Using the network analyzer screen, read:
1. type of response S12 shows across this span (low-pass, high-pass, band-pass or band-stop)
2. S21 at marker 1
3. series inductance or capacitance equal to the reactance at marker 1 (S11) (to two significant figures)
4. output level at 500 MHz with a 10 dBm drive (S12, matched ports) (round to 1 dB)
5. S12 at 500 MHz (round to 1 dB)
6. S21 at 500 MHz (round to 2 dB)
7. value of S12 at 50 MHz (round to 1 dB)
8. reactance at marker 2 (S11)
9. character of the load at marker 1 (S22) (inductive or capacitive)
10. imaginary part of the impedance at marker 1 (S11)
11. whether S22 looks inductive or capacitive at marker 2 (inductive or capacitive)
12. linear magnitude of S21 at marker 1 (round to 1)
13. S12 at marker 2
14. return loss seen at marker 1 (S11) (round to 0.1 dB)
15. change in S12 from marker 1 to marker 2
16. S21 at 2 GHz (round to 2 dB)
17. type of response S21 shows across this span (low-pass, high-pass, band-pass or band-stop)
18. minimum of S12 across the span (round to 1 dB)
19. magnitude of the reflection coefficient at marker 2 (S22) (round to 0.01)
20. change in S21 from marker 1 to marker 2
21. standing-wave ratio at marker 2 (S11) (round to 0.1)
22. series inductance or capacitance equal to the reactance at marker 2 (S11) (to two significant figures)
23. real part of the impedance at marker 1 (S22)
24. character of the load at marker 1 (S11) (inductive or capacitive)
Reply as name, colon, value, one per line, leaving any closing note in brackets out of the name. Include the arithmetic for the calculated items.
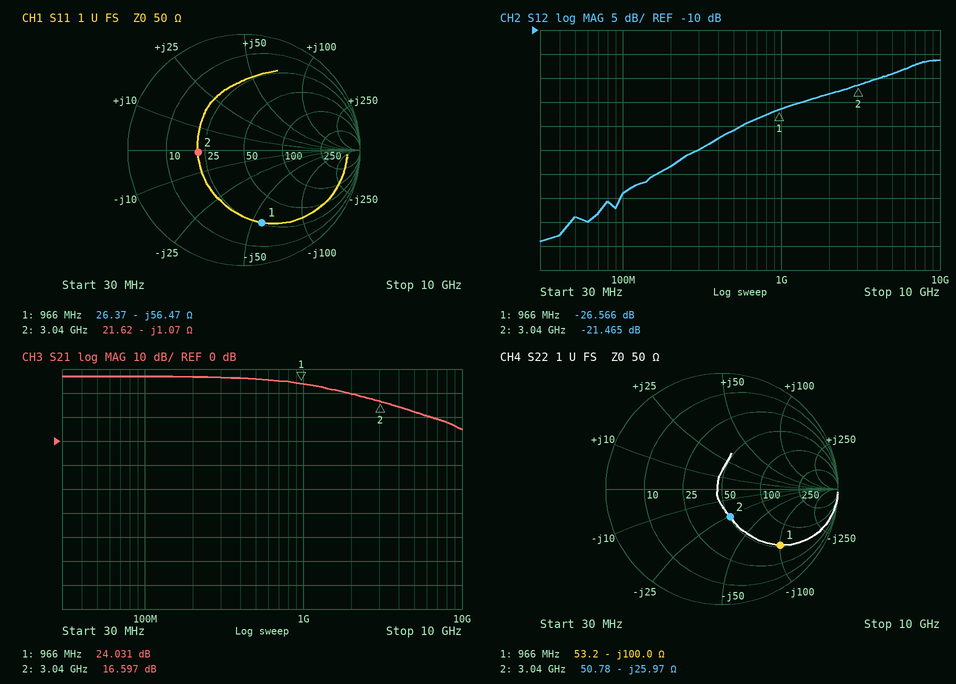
type of response S12 shows across this span: high-pass
S21 at marker 1: 24.031 dB
series inductance or capacitance equal to the reactance at marker 1 (S11): C = 1/(2π × 966 MHz × 56.47 Ω) ≈ 2.9 pF
output level at 500 MHz with a 10 dBm drive (S12, matched ports): 10 dBm + (-31 dB) = -21 dBm
S12 at 500 MHz: -31 dB
S21 at 500 MHz: 26 dB
value of S12 at 50 MHz: -49 dB
reactance at marker 2: -1.07 Ω
character of the load at marker 1 (S22): capacitive
imaginary part of the impedance at marker 1: -56.47 Ω
whether S22 looks inductive or capacitive at marker 2: capacitive
linear magnitude of S21 at marker 1: 10^(24.031/20) ≈ 16
S12 at marker 2: -21.465 dB
return loss seen at marker 1 (S11): 3.8 dB
change in S12 from marker 1 to marker 2: -21.465 − (-26.566) = 5.101 dB
S21 at 2 GHz: 20 dB
type of response S21 shows across this span: low-pass
minimum of S12 across the span: -54 dB
magnitude of the reflection coefficient at marker 2 (S22): 0.25
change in S21 from marker 1 to marker 2: 16.597 − (24.031) = -7.434 dB
standing-wave ratio at marker 2 (S11): 2.3
series inductance or capacitance equal to the reactance at marker 2 (S11): C = 1/(2π × 3.04 GHz × 1.07 Ω) ≈ 49 pF
real part of the impedance at marker 1: 53.2 Ω
character of the load at marker 1 (S11): capacitive
